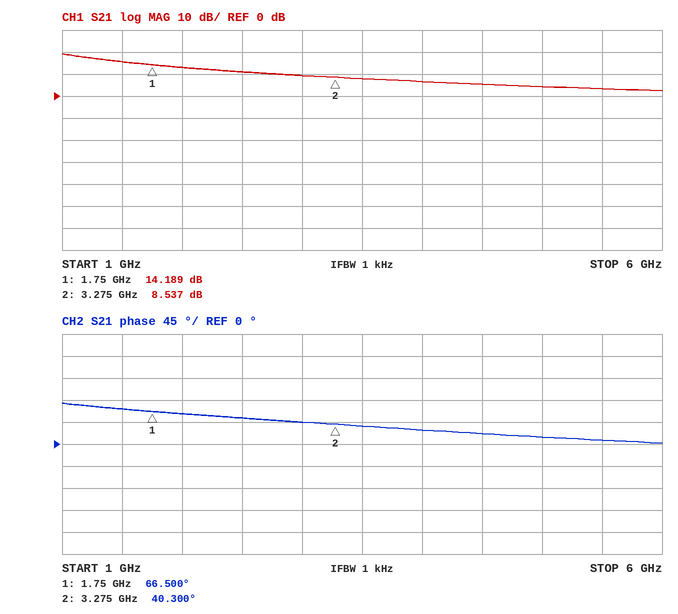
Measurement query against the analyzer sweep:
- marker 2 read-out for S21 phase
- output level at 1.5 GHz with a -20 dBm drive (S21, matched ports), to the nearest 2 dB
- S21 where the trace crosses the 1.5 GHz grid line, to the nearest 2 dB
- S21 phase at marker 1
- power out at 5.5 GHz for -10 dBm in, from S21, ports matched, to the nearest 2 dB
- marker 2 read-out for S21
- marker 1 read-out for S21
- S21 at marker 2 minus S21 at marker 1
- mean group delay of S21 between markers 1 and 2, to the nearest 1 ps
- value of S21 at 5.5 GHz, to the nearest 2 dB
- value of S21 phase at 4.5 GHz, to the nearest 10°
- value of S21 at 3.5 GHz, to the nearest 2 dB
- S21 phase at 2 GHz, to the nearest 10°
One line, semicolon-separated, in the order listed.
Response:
40.300°; -4 dBm; 16 dB; 66.500°; -6 dBm; 8.537 dB; 14.189 dB; -5.652 dB; 48 ps; 4 dB; 20°; 8 dB; 60°
